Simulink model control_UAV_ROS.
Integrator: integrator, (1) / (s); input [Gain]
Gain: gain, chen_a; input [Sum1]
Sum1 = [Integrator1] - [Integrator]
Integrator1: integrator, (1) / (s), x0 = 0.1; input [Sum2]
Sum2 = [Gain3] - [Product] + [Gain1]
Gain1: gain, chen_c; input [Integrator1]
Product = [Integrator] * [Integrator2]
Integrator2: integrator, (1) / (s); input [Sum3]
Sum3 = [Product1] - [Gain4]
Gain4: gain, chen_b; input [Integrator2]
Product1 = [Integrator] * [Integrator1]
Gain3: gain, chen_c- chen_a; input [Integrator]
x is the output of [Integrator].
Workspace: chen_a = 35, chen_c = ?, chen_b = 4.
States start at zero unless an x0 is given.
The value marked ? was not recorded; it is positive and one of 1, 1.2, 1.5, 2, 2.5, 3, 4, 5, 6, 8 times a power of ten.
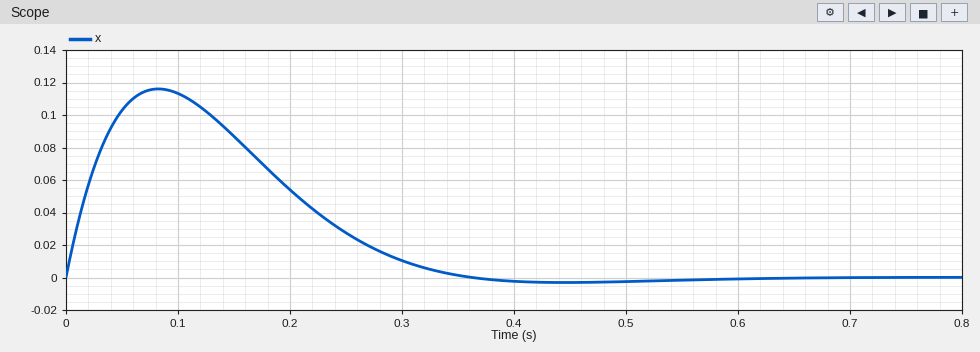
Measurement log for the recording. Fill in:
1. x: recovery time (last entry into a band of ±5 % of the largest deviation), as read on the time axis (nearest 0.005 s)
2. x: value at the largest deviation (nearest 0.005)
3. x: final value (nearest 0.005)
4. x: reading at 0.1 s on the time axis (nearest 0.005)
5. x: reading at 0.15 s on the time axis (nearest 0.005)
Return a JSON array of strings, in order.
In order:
["0.320 s", "0.115", "0.000", "0.115", "0.085"]
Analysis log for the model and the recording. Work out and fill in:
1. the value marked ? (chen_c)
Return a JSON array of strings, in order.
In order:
["15"]
